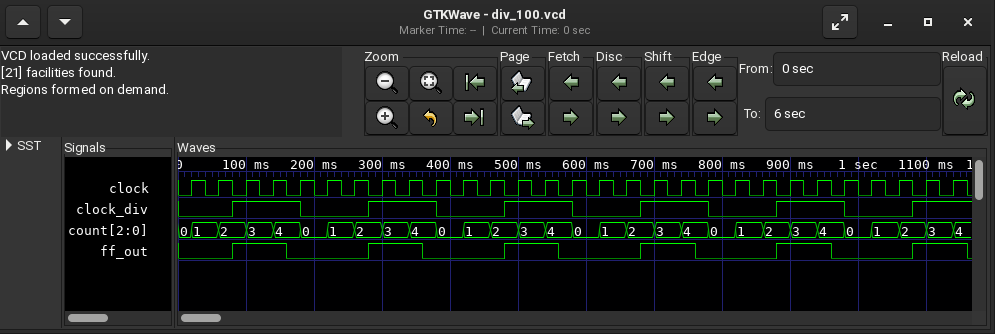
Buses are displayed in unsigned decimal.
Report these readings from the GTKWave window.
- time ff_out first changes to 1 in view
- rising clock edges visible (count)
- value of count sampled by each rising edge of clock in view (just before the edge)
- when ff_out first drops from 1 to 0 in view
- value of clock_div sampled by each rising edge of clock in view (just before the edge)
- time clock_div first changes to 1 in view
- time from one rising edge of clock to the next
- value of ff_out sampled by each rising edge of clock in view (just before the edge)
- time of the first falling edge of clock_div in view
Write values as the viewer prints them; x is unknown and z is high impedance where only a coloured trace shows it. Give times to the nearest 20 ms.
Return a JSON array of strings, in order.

["80 ms", "29", "0, 1, 2, 3, 4, 0, 1, 2, 3, 4, 0, 1, 2, 3, 4, 0, 1, 2, 3, 4, 0, 1, 2, 3, 4, 0, 1, 2, 3", "160 ms", "0 0 1 1 1 0 0 1 1 1 0 0 1 1 1 0 0 1 1 1 0 0 1 1 1 0 0 1 1", "80 ms", "40 ms", "0 0 1 1 0 0 0 1 1 0 0 0 1 1 0 0 0 1 1 0 0 0 1 1 0 0 0 1 1", "180 ms"]
